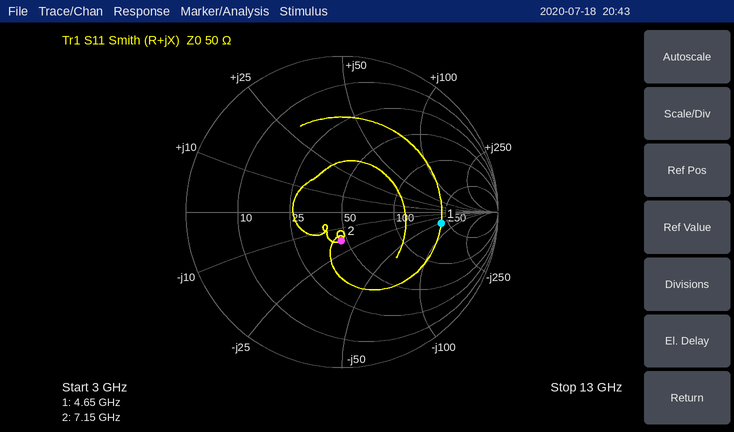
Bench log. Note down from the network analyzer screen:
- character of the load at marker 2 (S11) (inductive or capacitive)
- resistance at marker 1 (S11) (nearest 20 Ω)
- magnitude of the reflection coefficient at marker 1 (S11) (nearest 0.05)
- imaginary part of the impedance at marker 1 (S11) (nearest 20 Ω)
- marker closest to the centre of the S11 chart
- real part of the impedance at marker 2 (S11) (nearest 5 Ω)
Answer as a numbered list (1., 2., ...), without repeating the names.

1. capacitive
2. 220 Ω
3. 0.65
4. -60 Ω
5. marker 2
6. 45 Ω
